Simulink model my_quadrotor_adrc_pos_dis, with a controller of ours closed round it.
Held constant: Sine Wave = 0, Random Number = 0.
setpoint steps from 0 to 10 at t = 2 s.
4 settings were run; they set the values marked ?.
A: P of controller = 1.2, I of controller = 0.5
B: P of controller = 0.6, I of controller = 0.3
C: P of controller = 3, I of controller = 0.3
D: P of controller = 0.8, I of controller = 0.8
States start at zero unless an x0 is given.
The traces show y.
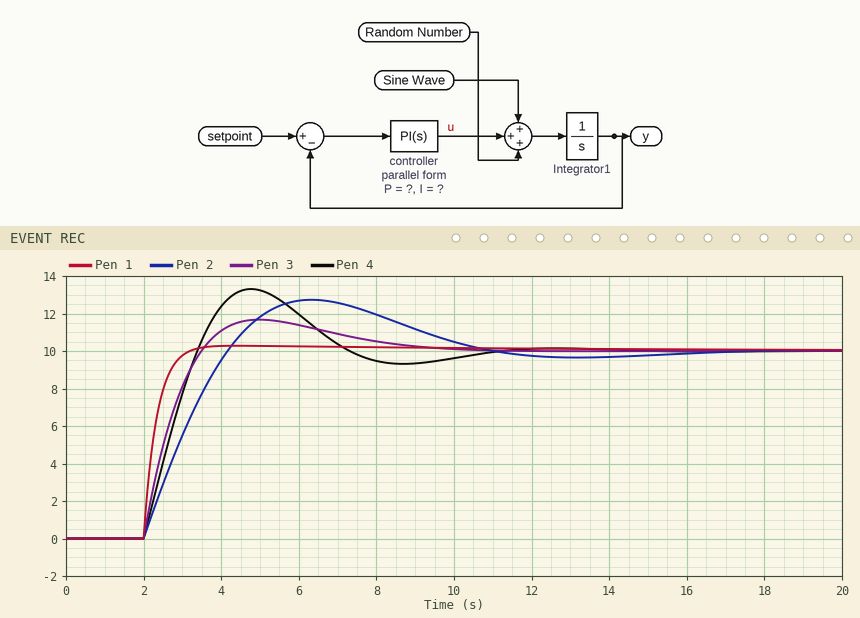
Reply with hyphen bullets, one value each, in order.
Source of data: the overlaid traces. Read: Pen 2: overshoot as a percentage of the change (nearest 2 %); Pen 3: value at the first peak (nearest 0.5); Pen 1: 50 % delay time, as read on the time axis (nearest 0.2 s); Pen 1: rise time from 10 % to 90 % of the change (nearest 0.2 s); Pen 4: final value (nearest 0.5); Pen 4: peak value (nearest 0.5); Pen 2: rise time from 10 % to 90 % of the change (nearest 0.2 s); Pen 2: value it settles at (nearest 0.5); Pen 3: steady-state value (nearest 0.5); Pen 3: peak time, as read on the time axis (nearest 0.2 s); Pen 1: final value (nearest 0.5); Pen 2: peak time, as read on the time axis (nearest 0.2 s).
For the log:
- 28 %
- 11.5
- 2.2 s
- 0.6 s
- 10.0
- 13.5
- 1.6 s
- 10.0
- 10.0
- 5.0 s
- 10.0
- 6.4 s
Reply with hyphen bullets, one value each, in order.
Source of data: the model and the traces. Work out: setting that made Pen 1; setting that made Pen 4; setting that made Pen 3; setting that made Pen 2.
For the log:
- C
- D
- A
- B
